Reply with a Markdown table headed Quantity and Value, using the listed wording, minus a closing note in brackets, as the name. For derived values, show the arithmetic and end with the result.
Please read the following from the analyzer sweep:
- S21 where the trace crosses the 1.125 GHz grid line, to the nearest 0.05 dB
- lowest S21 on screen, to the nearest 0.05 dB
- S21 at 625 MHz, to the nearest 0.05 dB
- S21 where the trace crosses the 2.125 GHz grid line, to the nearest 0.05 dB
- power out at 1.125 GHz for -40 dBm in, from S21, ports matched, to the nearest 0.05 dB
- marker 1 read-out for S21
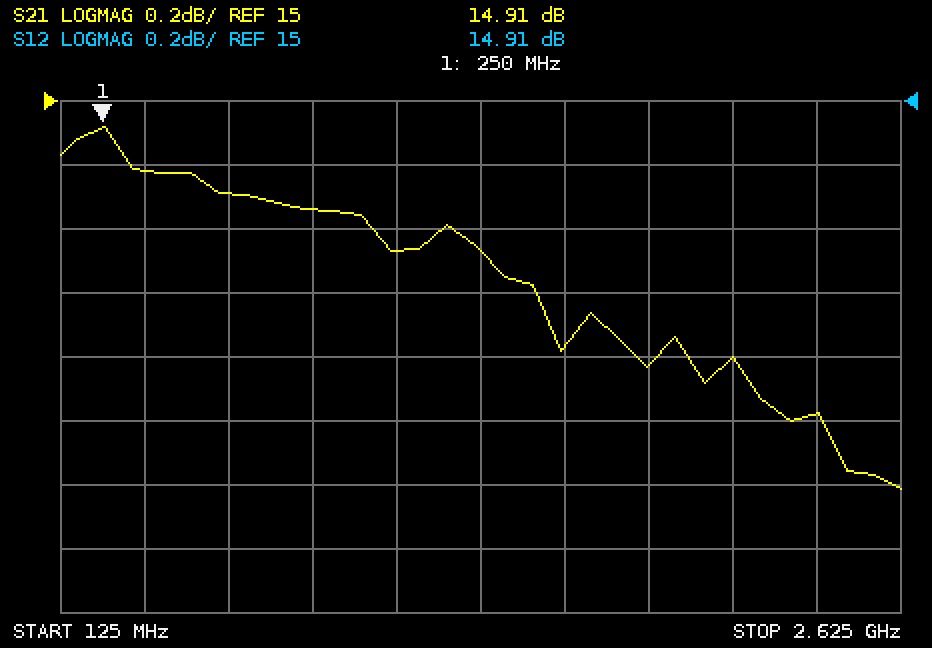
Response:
| Quantity | Value |
|---|---|
| S21 where the trace crosses the 1.125 GHz grid line, to the nearest 0.05 dB | 14.55 dB |
| lowest S21 on screen, to the nearest 0.05 dB | 13.80 dB |
| S21 at 625 MHz, to the nearest 0.05 dB | 14.70 dB |
| S21 where the trace crosses the 2.125 GHz grid line, to the nearest 0.05 dB | 14.20 dB |
| power out at 1.125 GHz for -40 dBm in, from S21, ports matched, to the nearest 0.05 dB | -40 dBm + (14.55 dB) = -25.45 dBm |
| marker 1 read-out for S21 | 14.91 dB |
